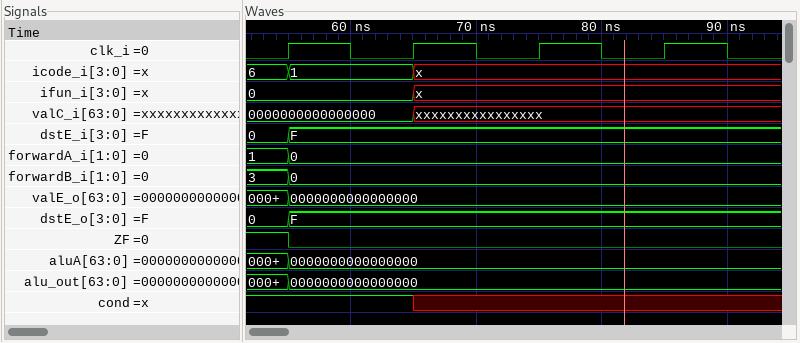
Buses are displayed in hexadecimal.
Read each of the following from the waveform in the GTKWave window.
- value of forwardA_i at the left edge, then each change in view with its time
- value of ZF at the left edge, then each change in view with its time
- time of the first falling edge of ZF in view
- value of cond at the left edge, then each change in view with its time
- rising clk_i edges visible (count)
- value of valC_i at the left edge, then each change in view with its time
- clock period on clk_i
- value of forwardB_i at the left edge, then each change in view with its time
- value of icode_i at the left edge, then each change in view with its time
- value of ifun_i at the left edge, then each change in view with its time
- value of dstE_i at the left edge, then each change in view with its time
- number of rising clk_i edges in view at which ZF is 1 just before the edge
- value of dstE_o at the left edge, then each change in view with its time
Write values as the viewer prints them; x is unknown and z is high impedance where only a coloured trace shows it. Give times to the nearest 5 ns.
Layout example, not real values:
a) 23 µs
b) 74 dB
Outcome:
a) 1, 0 at 55 ns
b) 1, 0 at 55 ns
c) 55 ns
d) 1, x at 65 ns
e) 4
f) 0000000000000000, xxxxxxxxxxxxxxxx at 65 ns
g) 10 ns
h) 3, 0 at 55 ns
i) 6, 1 at 55 ns, x at 65 ns
j) 0, x at 65 ns
k) 0, F at 55 ns
l) 1
m) 0, F at 55 ns
